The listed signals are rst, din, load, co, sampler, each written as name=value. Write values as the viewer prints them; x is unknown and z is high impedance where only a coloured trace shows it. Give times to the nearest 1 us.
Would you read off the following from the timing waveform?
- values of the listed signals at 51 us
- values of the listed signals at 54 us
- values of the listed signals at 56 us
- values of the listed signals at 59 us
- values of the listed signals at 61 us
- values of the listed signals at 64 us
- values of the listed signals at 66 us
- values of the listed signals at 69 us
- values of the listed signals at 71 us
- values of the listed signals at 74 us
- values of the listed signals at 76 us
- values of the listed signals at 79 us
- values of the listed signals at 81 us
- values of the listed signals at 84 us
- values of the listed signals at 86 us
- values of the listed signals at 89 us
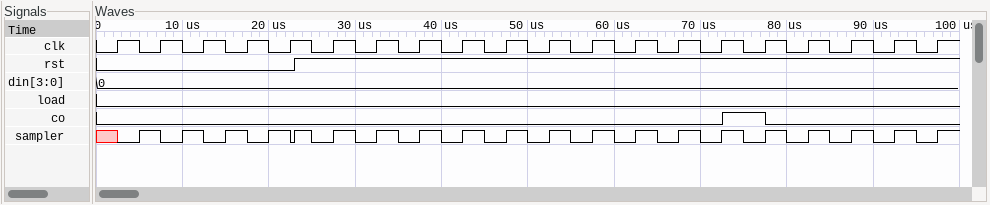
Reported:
rst=1, din=0, load=0, co=0, sampler=0
rst=1, din=0, load=0, co=0, sampler=1
rst=1, din=0, load=0, co=0, sampler=0
rst=1, din=0, load=0, co=0, sampler=1
rst=1, din=0, load=0, co=0, sampler=0
rst=1, din=0, load=0, co=0, sampler=1
rst=1, din=0, load=0, co=0, sampler=0
rst=1, din=0, load=0, co=0, sampler=1
rst=1, din=0, load=0, co=0, sampler=0
rst=1, din=0, load=0, co=1, sampler=1
rst=1, din=0, load=0, co=1, sampler=0
rst=1, din=0, load=0, co=0, sampler=1
rst=1, din=0, load=0, co=0, sampler=0
rst=1, din=0, load=0, co=0, sampler=1
rst=1, din=0, load=0, co=0, sampler=0
rst=1, din=0, load=0, co=0, sampler=1
